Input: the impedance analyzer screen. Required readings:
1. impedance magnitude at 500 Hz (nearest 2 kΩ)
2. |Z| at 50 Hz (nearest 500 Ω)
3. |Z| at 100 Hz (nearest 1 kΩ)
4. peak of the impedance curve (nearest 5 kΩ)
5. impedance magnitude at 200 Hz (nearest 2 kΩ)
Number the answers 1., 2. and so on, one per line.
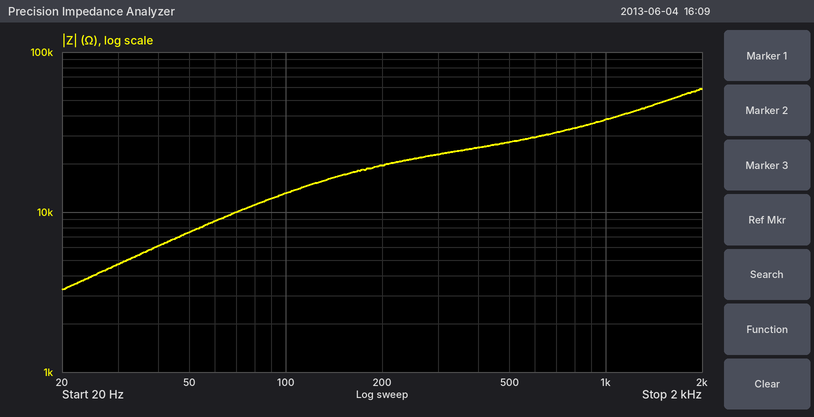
1. 28 kΩ
2. 7.5 kΩ
3. 13 kΩ
4. 60 kΩ
5. 20 kΩ
